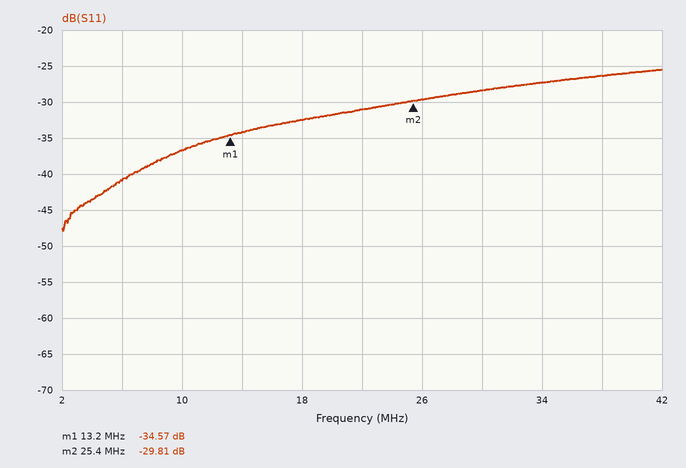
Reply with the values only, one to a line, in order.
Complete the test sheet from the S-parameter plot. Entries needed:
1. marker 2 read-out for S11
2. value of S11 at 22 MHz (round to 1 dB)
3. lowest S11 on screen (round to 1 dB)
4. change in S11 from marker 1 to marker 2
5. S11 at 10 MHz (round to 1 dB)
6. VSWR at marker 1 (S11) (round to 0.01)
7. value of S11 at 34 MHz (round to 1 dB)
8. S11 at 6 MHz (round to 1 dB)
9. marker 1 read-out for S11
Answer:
-29.81 dB
-31 dB
-48 dB
4.76 dB
-37 dB
1.04
-27 dB
-41 dB
-34.57 dB
